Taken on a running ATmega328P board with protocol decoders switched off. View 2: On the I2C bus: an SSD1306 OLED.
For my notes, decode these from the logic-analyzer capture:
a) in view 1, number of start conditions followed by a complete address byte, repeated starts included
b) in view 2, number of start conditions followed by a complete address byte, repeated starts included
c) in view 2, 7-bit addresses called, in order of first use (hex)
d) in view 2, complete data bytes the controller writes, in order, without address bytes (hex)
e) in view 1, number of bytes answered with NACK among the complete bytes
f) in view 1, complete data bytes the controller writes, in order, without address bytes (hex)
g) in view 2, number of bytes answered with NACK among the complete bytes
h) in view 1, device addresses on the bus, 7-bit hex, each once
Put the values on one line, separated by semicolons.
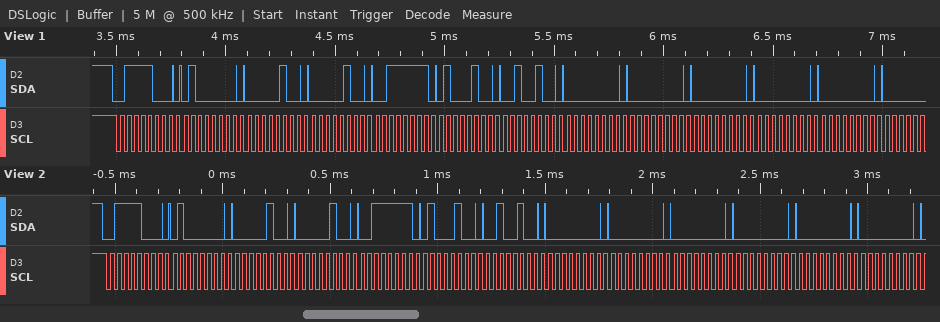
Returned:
1; 1; 0x3C; 40 04 04 3F 44 24 00 00 00 00 00 00; 0; 40 04 04 3F 44 24 00 00 00 00 00; 0; 0x3C
